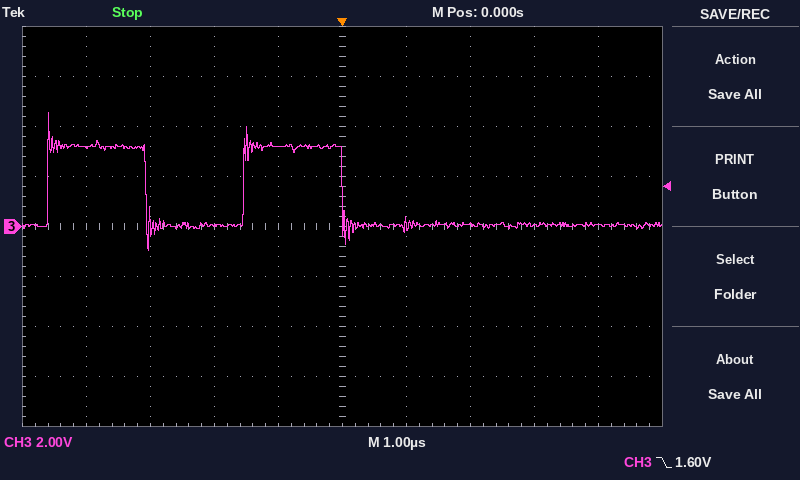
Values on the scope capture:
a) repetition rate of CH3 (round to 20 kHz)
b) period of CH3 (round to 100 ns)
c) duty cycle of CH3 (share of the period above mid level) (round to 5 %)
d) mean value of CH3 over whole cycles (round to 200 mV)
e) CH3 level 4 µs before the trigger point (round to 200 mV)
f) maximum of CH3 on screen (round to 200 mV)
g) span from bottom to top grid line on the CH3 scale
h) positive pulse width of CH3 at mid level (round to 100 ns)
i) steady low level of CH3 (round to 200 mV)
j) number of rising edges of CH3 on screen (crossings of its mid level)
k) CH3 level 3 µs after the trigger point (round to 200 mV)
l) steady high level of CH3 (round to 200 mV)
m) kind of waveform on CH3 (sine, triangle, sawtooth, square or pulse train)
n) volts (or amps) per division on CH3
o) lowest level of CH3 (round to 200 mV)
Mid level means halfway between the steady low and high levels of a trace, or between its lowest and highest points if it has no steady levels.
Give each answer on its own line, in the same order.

320 kHz
3.1 µs
50 %
1.6 V
3.2 V
4.6 V
16 V
1.5 µs
0.0 V
2
0.0 V
3.2 V
square
2 V
-1.0 V
